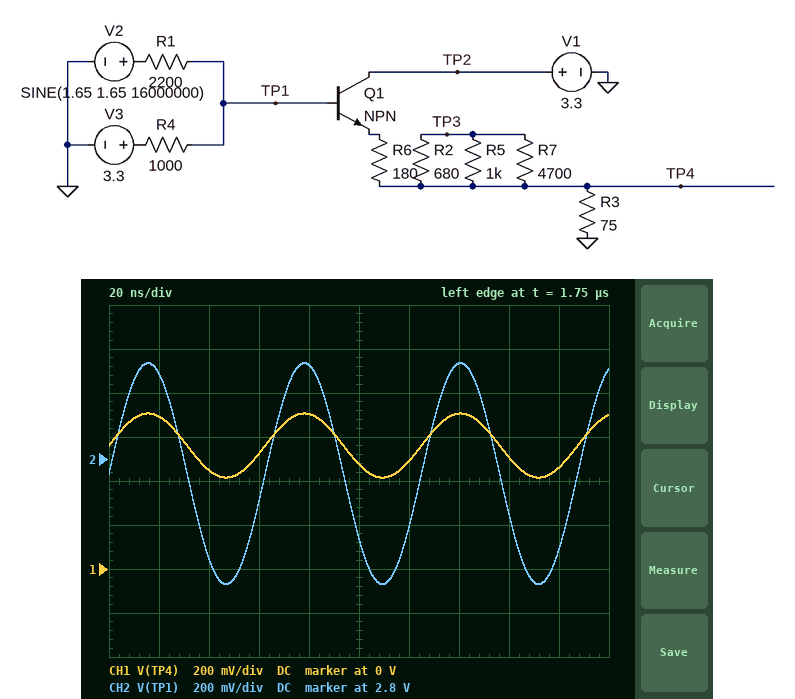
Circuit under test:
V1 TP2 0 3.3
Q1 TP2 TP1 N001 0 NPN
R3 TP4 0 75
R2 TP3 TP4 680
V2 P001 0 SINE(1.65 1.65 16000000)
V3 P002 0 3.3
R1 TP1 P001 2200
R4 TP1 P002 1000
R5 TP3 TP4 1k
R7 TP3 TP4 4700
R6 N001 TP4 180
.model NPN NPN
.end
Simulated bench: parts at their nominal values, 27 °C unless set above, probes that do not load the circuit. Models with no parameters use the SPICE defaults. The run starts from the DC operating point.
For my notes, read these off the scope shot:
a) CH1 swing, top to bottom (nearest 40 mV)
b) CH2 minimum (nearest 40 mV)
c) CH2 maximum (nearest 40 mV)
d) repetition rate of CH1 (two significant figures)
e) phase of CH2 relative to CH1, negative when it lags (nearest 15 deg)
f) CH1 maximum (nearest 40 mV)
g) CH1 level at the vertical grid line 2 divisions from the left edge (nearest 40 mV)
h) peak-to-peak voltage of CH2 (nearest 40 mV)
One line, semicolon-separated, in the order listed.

280 mV; 2.24 V; 3.24 V; 16 MHz; 0 deg; 720 mV; 440 mV; 1.00 V
